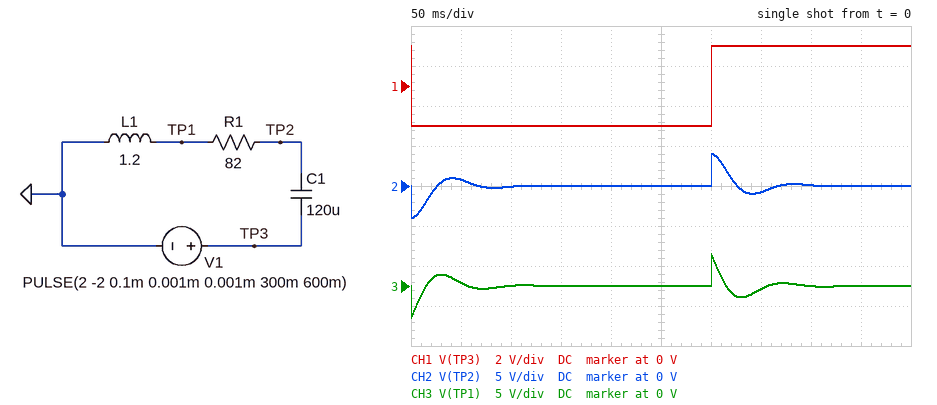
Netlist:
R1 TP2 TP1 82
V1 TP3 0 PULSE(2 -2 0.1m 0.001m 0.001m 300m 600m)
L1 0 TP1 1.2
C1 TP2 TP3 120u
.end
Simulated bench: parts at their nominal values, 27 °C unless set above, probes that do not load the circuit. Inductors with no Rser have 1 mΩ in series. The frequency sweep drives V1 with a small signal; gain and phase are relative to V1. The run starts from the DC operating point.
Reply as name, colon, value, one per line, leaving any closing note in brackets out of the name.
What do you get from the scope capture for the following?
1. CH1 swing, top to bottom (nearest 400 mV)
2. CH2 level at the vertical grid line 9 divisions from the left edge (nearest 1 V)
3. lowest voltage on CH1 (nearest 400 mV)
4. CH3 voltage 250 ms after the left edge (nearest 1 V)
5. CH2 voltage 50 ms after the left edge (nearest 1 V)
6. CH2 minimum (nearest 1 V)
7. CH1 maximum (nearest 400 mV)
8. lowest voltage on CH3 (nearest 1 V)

CH1 swing, top to bottom: 4.0 V
CH2 level at the vertical grid line 9 divisions from the left edge: 0 V
lowest voltage on CH1: -2.0 V
CH3 voltage 250 ms after the left edge: 0 V
CH2 voltage 50 ms after the left edge: 1 V
CH2 minimum: -4 V
CH1 maximum: 2.0 V
lowest voltage on CH3: -4 V
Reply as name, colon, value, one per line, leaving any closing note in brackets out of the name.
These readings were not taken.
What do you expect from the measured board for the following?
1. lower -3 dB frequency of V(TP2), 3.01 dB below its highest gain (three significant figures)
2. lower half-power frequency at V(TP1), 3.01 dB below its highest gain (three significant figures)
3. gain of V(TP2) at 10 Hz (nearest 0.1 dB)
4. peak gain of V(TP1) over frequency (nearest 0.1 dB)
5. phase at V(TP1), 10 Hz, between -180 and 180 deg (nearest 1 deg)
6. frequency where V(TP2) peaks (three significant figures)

lower -3 dB frequency of V(TP2), 3.01 dB below its highest gain: 10.2 Hz
lower half-power frequency at V(TP1), 3.01 dB below its highest gain: 11.2 Hz
gain of V(TP2) at 10 Hz: 0.9 dB
peak gain of V(TP1) over frequency: 2.5 dB
phase at V(TP1), 10 Hz, between -180 and 180 deg: 125 deg
frequency where V(TP2) peaks: 14.9 Hz
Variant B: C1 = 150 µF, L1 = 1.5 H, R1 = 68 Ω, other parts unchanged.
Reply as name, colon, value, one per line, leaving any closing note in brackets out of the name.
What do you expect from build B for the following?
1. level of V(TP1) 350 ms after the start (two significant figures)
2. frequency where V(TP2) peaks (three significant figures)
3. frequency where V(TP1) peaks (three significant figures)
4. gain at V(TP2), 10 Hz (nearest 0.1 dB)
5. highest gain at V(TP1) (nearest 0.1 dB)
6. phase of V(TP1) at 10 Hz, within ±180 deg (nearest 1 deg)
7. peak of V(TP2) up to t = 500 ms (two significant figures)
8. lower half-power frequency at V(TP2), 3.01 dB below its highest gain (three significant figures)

level of V(TP1) 350 ms after the start: -1.3 V
frequency where V(TP2) peaks: 11.6 Hz
frequency where V(TP1) peaks: 12.1 Hz
gain at V(TP2), 10 Hz: 4.5 dB
highest gain at V(TP1): 3.9 dB
phase of V(TP1) at 10 Hz, within ±180 deg: 100 deg
peak of V(TP2) up to t = 500 ms: 4.0 V
lower half-power frequency at V(TP2), 3.01 dB below its highest gain: 8.51 Hz
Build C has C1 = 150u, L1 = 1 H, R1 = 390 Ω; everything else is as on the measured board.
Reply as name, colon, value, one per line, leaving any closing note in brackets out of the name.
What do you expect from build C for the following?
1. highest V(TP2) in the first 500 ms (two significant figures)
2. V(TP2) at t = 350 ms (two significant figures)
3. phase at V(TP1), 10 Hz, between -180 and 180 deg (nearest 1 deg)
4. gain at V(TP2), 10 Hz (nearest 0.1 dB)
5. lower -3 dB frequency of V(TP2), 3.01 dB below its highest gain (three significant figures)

highest V(TP2) in the first 500 ms: 4.0 V
V(TP2) at t = 350 ms: 1.7 V
phase at V(TP1), 10 Hz, between -180 and 180 deg: 96 deg
gain at V(TP2), 10 Hz: 0.1 dB
lower -3 dB frequency of V(TP2), 3.01 dB below its highest gain: 2.78 Hz
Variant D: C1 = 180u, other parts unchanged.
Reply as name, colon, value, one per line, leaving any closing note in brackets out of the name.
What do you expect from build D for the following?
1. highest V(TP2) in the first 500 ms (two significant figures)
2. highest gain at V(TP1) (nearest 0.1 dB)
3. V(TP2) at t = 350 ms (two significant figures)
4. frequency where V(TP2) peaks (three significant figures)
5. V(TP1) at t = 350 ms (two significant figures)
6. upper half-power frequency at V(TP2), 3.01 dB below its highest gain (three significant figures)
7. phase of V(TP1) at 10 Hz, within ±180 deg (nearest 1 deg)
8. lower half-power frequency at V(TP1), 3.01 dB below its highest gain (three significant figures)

highest V(TP2) in the first 500 ms: 4.0 V
highest gain at V(TP1): 1.2 dB
V(TP2) at t = 350 ms: -630 mV
frequency where V(TP2) peaks: 12.7 Hz
V(TP1) at t = 350 ms: -800 mV
upper half-power frequency at V(TP2), 3.01 dB below its highest gain: 57.2 Hz
phase of V(TP1) at 10 Hz, within ±180 deg: 99 deg
lower half-power frequency at V(TP1), 3.01 dB below its highest gain: 9.27 Hz
